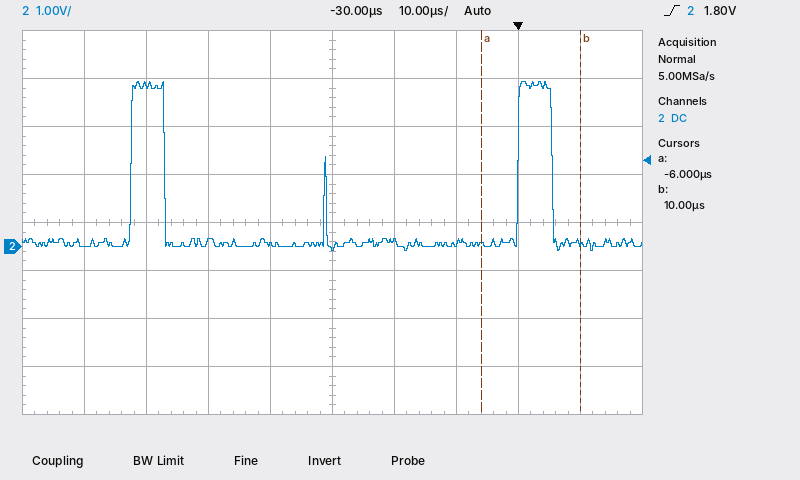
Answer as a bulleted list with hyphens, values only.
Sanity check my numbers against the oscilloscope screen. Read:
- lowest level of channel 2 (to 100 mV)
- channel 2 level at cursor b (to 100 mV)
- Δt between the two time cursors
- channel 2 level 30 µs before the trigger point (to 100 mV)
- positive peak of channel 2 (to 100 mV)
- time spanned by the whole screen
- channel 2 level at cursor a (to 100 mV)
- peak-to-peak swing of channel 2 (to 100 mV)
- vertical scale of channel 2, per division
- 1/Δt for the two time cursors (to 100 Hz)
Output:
- -100 mV
- 100 mV
- 16 µs
- 0.0 V
- 3.4 V
- 100 µs
- 0.0 V
- 3.5 V
- 1 V
- 62.5 kHz
